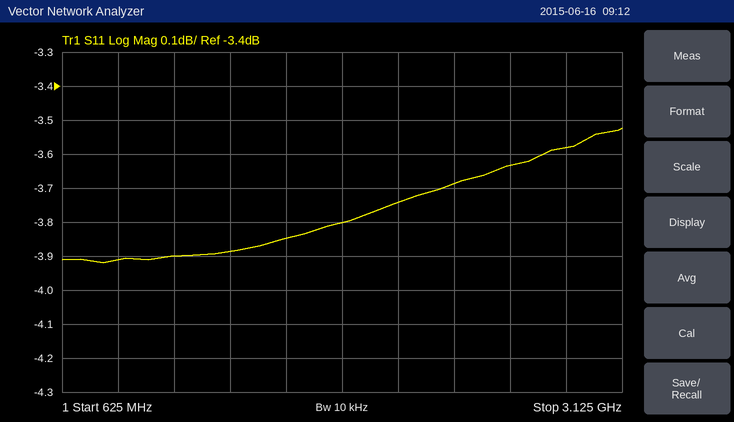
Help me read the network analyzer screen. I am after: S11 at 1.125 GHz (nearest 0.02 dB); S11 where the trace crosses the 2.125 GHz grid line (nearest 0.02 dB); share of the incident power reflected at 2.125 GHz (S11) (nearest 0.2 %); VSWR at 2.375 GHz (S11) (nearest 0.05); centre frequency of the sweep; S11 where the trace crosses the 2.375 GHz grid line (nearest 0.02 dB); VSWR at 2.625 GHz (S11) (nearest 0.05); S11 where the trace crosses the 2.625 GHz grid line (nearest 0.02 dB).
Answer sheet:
-3.90 dB
-3.74 dB
42.2 %
4.80
1.875 GHz
-3.68 dB
4.85
-3.64 dB
